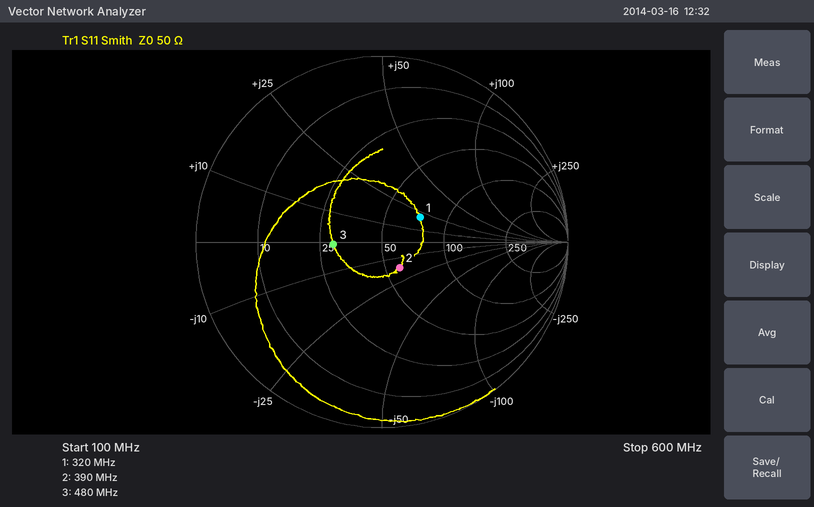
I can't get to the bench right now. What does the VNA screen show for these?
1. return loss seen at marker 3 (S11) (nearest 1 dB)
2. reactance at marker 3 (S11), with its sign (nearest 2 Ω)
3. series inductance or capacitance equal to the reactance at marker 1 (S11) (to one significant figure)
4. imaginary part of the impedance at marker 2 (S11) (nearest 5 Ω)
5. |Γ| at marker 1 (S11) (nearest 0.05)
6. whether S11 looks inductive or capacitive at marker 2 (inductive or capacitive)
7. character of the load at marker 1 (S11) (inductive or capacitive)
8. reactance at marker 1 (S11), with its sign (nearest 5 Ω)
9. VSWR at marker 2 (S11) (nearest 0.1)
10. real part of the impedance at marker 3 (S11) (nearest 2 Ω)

12 dB
0 Ω
10 nH
-15 Ω
0.25
capacitive
inductive
+20 Ω
1.4
30 Ω
